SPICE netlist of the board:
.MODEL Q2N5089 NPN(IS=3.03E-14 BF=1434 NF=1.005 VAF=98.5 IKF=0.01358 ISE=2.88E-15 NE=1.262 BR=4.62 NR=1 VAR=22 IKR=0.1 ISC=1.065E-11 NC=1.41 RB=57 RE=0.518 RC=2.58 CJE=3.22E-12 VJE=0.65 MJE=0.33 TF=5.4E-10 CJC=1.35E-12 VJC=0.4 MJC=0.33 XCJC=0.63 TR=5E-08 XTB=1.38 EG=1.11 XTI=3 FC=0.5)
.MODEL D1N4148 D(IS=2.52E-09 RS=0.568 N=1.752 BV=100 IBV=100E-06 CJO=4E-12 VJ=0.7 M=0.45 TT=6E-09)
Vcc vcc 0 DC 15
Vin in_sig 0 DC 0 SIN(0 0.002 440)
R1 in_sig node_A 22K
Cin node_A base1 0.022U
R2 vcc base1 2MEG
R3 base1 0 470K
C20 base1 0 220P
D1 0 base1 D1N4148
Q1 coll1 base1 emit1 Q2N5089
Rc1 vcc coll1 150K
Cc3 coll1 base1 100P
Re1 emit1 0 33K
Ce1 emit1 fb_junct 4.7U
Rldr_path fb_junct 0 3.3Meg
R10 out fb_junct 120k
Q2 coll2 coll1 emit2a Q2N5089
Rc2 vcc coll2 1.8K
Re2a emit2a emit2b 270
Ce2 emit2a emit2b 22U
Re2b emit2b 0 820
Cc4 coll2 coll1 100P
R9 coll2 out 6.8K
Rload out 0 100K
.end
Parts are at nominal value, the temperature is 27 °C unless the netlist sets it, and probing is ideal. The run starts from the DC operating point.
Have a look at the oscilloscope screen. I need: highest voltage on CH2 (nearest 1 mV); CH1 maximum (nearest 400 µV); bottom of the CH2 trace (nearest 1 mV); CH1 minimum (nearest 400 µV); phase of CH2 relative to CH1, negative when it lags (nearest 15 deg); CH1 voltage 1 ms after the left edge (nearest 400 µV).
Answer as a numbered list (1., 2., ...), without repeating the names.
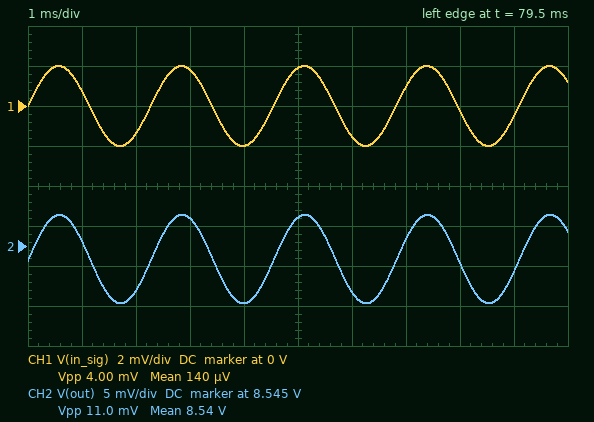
1. 8.549 V
2. 2.0 mV
3. 8.538 V
4. -2.0 mV
5. 0 deg
6. 800 µV
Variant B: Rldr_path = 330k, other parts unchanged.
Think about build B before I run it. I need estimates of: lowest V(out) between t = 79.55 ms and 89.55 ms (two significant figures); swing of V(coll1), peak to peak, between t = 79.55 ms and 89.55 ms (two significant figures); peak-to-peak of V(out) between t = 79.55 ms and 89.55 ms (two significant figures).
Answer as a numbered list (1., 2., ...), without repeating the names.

1. 8.4 V
2. 6.2 mV
3. 12 mV
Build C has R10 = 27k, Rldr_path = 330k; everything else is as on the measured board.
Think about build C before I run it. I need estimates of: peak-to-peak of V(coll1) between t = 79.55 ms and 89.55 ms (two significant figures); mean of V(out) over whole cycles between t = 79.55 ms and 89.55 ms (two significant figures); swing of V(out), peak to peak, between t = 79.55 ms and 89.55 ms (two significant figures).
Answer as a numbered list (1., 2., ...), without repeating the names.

1. 3.5 mV
2. 8.4 V
3. 6.2 mV
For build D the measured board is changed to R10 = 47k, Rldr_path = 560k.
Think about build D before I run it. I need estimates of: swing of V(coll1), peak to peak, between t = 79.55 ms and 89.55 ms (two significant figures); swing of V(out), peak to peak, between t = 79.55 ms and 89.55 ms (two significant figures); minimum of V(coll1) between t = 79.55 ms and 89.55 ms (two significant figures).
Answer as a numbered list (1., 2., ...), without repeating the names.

1. 4.1 mV
2. 7.6 mV
3. 4.1 V
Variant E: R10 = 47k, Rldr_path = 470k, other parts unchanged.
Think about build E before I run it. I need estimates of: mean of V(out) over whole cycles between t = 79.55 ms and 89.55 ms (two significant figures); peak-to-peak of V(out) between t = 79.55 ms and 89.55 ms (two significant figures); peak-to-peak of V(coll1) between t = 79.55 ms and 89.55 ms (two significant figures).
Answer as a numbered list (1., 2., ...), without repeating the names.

1. 8.4 V
2. 7.6 mV
3. 4.2 mV
